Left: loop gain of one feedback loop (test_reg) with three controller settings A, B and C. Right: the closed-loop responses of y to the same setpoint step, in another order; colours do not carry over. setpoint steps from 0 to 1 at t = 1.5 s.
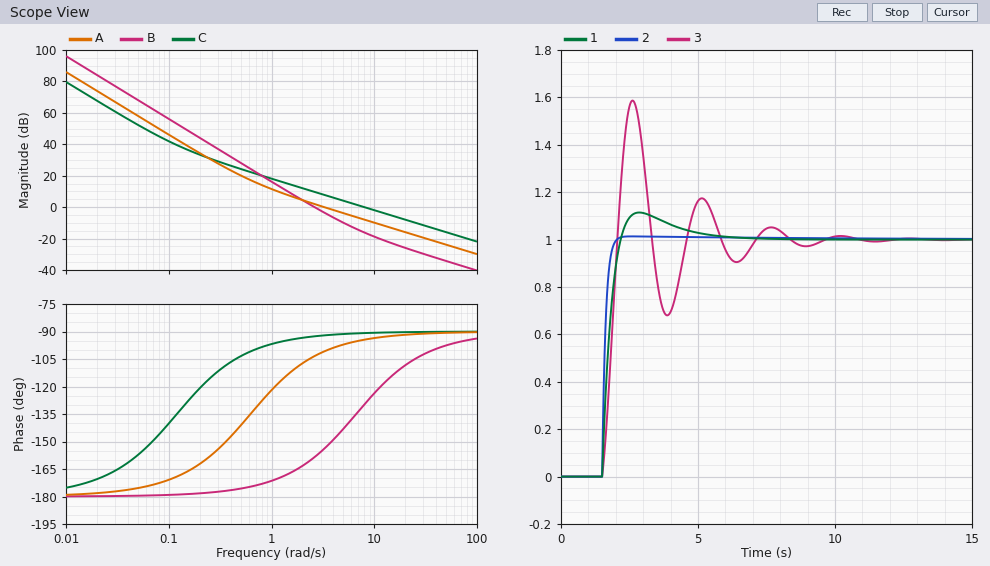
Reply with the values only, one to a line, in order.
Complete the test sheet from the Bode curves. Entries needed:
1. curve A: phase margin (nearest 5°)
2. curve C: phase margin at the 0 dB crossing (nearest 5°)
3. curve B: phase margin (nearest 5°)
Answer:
80°
90°
20°
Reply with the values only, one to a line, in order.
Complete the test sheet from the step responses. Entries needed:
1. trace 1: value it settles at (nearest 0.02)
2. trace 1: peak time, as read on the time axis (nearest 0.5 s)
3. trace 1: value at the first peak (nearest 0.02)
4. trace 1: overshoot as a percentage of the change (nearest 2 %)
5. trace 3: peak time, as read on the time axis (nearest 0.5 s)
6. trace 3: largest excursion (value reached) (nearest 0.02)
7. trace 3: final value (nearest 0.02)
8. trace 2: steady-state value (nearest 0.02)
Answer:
1.00
3.0 s
1.12
12 %
2.5 s
1.58
1.00
1.00
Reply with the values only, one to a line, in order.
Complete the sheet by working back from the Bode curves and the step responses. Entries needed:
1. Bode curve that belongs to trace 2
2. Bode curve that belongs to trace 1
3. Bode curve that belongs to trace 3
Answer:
C
A
B
